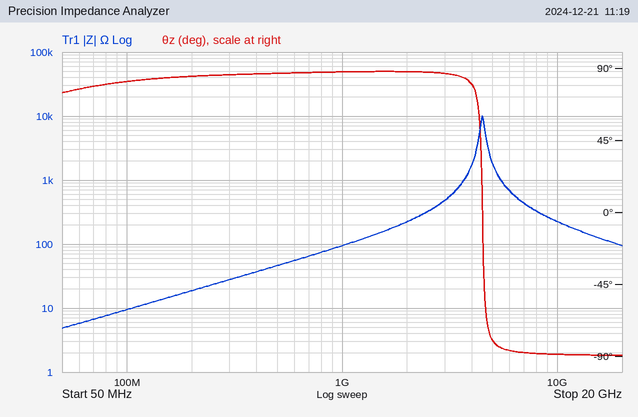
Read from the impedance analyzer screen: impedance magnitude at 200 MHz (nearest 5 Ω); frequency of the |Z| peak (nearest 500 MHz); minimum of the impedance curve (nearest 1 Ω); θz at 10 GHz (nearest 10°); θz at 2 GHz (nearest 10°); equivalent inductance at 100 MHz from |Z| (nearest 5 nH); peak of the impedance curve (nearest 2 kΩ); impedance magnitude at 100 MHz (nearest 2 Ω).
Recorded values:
20 Ω
4.5 GHz
5 Ω
-90°
90°
15 nH
10 kΩ
10 Ω
